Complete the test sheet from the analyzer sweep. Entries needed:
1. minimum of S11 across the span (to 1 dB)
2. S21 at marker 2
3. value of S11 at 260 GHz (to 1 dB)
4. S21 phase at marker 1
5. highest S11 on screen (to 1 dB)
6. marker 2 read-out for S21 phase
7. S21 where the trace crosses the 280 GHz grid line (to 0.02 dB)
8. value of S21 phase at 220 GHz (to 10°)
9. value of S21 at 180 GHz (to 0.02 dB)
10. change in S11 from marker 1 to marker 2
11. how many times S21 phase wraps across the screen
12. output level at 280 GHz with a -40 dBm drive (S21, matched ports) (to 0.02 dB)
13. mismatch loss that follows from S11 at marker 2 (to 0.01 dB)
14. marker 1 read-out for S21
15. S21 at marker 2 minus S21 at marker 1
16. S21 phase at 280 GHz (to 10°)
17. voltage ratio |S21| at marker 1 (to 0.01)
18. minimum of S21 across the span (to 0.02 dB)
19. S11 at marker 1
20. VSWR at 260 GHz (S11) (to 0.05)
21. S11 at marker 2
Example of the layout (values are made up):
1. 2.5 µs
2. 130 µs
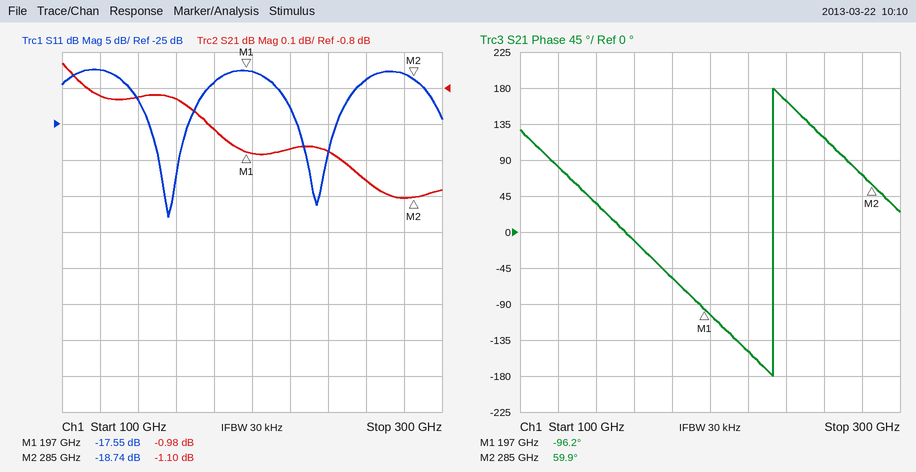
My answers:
1. -38 dB
2. -1.10 dB
3. -19 dB
4. -96.2°
5. -17 dB
6. 59.9°
7. -1.10 dB
8. -150°
9. -0.92 dB
10. -1.19 dB
11. 1
12. -41.10 dBm
13. 0.06 dB
14. -0.98 dB
15. -0.12 dB
16. 70°
17. 0.89
18. -1.10 dB
19. -17.55 dB
20. 1.25
21. -18.74 dB
